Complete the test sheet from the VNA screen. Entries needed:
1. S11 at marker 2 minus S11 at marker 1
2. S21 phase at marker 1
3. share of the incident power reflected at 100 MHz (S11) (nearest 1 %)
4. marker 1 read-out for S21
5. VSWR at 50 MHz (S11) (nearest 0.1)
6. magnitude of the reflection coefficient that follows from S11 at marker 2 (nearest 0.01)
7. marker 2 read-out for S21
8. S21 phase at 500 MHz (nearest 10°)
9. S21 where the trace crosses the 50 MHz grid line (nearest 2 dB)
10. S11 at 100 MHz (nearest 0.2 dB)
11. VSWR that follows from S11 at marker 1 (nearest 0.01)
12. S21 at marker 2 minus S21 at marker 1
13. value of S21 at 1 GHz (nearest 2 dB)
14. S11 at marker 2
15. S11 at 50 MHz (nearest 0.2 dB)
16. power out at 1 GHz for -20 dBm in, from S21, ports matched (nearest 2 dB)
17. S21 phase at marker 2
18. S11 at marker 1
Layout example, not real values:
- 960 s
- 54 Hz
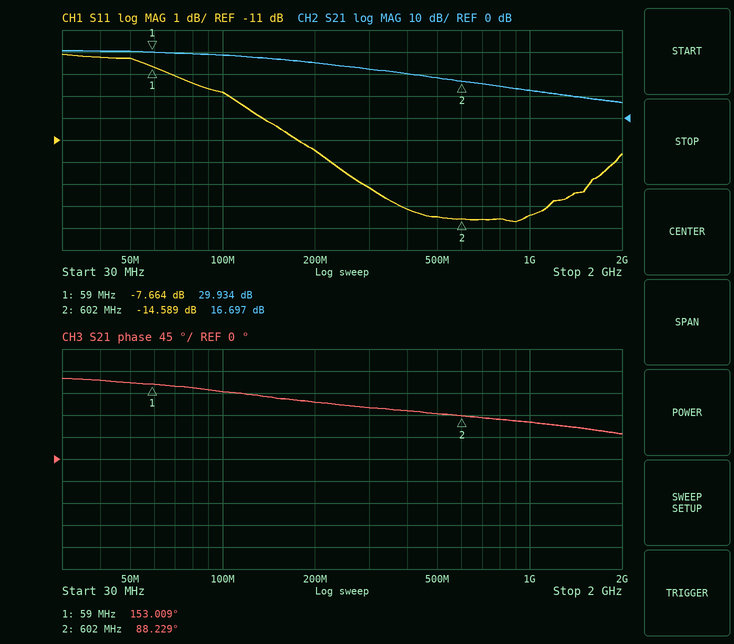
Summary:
- -6.925 dB
- 153.009°
- 13 %
- 29.934 dB
- 2.5
- 0.19
- 16.697 dB
- 90°
- 30 dB
- -8.8 dB
- 2.41
- -13.237 dB
- 12 dB
- -14.589 dB
- -7.2 dB
- -8 dBm
- 88.229°
- -7.664 dB
